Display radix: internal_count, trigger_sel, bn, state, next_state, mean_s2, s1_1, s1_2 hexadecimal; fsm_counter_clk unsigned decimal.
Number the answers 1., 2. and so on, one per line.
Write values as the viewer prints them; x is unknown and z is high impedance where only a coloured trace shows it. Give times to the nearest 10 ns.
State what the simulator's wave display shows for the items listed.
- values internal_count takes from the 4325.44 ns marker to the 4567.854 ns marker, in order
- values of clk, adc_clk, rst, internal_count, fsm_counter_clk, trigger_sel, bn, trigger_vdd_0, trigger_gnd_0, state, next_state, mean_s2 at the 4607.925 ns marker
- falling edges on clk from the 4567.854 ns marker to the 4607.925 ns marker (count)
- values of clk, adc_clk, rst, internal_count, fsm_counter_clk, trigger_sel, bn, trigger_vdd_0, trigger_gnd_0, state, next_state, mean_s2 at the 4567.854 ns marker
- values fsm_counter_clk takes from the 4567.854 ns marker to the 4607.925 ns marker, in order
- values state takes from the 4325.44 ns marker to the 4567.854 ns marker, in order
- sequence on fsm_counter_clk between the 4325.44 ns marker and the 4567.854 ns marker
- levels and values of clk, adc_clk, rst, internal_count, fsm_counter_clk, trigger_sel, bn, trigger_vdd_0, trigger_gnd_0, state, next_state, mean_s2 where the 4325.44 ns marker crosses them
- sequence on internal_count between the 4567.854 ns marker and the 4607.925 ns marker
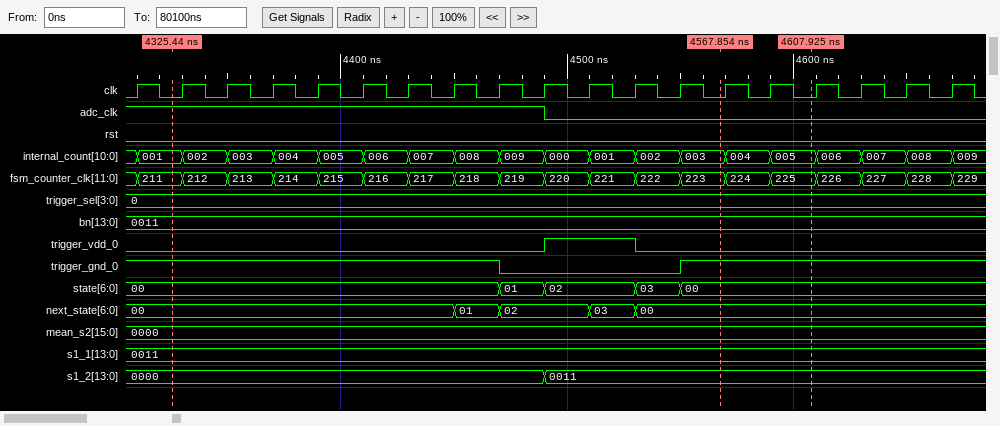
1. 001, 002, 003, 004, 005, 006, 007, 008, 009, 000, 001, 002, 003
2. clk=0, adc_clk=0, rst=0, internal_count=005, fsm_counter_clk=225, trigger_sel=0, bn=0011, trigger_vdd_0=0, trigger_gnd_0=1, state=00, next_state=00, mean_s2=0000
3. 2
4. clk=0, adc_clk=0, rst=0, internal_count=003, fsm_counter_clk=223, trigger_sel=0, bn=0011, trigger_vdd_0=0, trigger_gnd_0=1, state=00, next_state=00, mean_s2=0000
5. 223, 224, 225
6. 00, 01, 02, 03, 00
7. 211, 212, 213, 214, 215, 216, 217, 218, 219, 220, 221, 222, 223
8. clk=0, adc_clk=1, rst=0, internal_count=001, fsm_counter_clk=211, trigger_sel=0, bn=0011, trigger_vdd_0=0, trigger_gnd_0=1, state=00, next_state=00, mean_s2=0000
9. 003, 004, 005
